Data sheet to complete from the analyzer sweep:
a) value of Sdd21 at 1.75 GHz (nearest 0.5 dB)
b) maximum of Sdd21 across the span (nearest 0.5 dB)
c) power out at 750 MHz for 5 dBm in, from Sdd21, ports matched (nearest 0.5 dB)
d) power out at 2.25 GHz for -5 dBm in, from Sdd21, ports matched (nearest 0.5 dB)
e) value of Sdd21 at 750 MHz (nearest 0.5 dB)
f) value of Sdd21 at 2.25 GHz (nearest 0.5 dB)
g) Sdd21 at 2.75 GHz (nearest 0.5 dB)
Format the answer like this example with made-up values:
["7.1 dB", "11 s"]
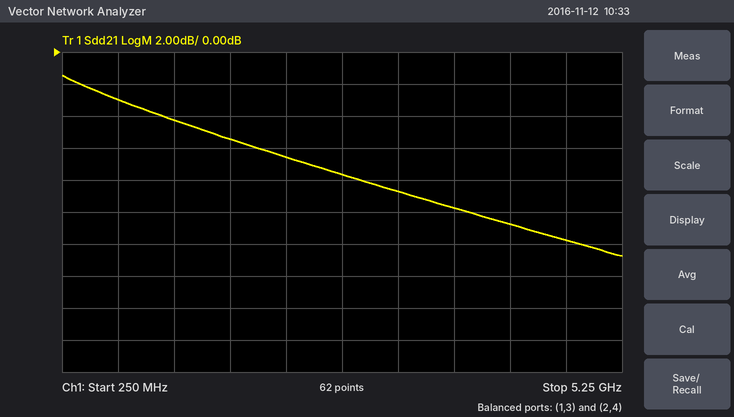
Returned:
["-5.5 dB", "-1.5 dB", "2.0 dBm", "-11.5 dBm", "-3.0 dB", "-6.5 dB", "-7.5 dB"]
